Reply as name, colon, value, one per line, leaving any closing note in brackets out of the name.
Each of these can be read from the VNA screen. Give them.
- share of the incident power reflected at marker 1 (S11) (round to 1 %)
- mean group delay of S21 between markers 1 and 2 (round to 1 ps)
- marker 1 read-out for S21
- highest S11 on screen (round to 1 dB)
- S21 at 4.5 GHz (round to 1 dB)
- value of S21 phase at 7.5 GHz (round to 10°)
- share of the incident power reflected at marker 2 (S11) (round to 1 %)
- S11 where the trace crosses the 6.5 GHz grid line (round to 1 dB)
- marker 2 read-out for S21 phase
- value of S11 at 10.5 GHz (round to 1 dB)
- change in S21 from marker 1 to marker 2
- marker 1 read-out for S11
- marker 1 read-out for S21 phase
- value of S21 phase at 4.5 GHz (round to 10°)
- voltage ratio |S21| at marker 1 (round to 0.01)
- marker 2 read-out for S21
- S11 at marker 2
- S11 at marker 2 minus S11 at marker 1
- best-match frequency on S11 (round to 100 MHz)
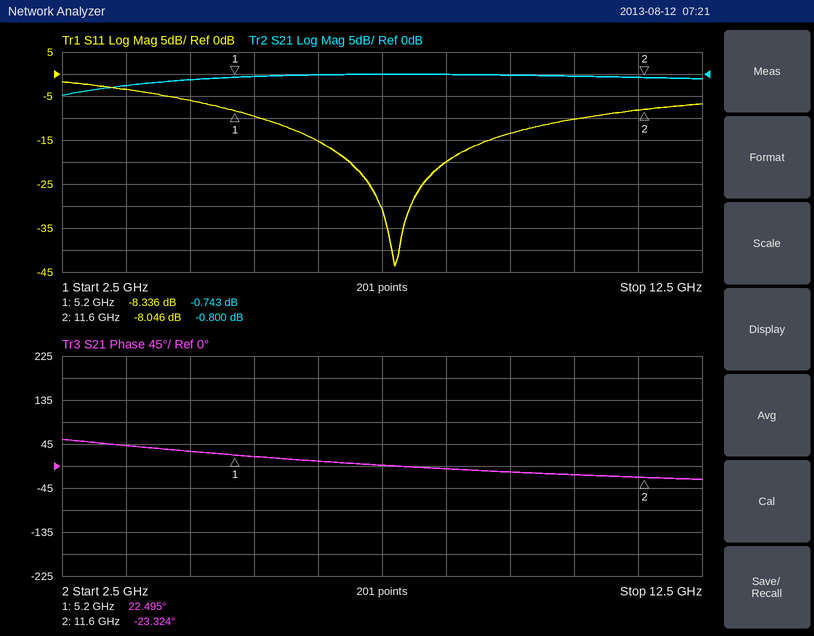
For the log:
share of the incident power reflected at marker 1 (S11): 15 %
mean group delay of S21 between markers 1 and 2: 20 ps
marker 1 read-out for S21: -0.743 dB
highest S11 on screen: -2 dB
S21 at 4.5 GHz: -1 dB
value of S21 phase at 7.5 GHz: 0°
share of the incident power reflected at marker 2 (S11): 16 %
S11 where the trace crosses the 6.5 GHz grid line: -15 dB
marker 2 read-out for S21 phase: -23.324°
value of S11 at 10.5 GHz: -10 dB
change in S21 from marker 1 to marker 2: -0.057 dB
marker 1 read-out for S11: -8.336 dB
marker 1 read-out for S21 phase: 22.495°
value of S21 phase at 4.5 GHz: 30°
voltage ratio |S21| at marker 1: 0.92
marker 2 read-out for S21: -0.800 dB
S11 at marker 2: -8.046 dB
S11 at marker 2 minus S11 at marker 1: 0.290 dB
best-match frequency on S11: 7.7 GHz
